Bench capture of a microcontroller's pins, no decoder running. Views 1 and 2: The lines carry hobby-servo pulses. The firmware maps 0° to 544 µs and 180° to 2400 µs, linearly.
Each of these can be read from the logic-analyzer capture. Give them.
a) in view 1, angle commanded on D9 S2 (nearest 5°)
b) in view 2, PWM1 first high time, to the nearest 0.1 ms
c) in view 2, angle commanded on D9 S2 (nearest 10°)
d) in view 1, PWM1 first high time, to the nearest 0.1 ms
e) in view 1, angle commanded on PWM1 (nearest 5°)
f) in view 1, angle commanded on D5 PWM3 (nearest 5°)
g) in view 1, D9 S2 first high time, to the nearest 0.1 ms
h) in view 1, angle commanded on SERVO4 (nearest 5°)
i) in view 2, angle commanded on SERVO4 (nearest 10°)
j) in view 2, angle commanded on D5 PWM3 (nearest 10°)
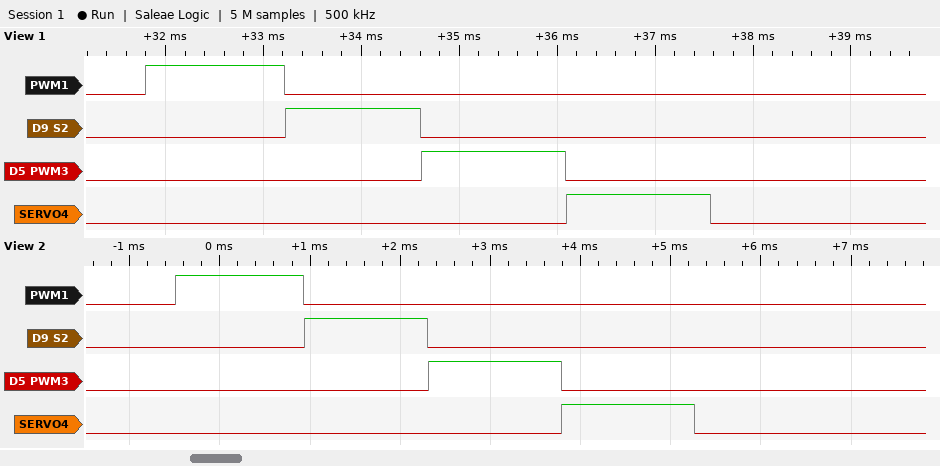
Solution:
80°
1.4 ms
80°
1.4 ms
85°
90°
1.4 ms
90°
90°
90°
